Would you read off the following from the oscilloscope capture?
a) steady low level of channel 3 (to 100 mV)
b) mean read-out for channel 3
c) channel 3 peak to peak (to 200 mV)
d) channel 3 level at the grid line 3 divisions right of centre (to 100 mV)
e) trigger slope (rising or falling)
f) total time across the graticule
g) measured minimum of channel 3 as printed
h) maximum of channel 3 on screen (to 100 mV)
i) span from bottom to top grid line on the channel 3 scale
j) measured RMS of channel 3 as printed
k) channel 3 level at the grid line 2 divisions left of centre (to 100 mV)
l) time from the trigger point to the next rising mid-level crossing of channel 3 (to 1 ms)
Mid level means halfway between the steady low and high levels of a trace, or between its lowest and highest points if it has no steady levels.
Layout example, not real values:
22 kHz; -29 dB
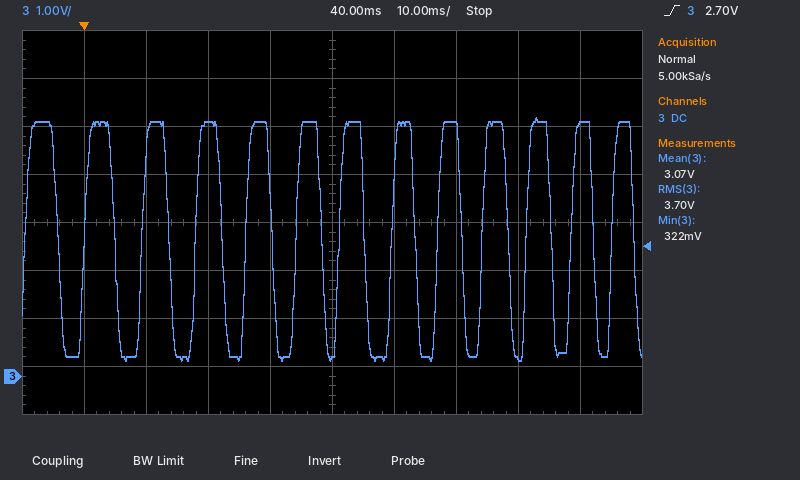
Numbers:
400 mV; 3.07 V; 5.0 V; 400 mV; rising; 100 ms; 322 mV; 5.4 V; 8 V; 3.70 V; 5.3 V; 9 ms
